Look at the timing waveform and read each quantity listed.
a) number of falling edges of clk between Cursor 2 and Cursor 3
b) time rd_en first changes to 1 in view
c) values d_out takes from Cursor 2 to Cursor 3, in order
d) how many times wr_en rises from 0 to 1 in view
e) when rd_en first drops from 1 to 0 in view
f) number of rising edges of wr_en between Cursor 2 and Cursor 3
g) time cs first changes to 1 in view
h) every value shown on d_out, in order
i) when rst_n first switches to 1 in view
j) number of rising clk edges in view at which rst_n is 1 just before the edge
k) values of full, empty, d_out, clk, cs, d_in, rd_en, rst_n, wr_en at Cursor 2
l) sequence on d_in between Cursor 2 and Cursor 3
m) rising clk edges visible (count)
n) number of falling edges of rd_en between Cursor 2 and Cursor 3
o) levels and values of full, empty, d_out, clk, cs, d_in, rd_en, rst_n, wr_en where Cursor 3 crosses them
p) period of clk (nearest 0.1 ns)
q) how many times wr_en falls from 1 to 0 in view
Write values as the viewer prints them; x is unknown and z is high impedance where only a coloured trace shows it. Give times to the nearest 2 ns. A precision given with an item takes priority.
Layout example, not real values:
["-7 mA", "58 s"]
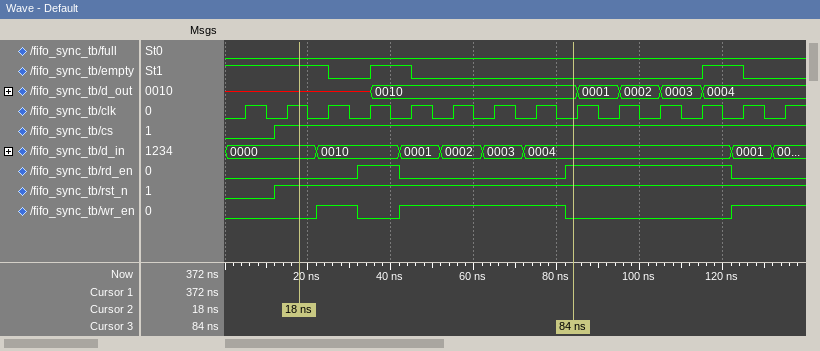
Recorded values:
["7", "32 ns", "x, 0010", "3", "42 ns", "2", "12 ns", "x, 0010, 0001, 0002, 0003, 0004", "12 ns", "13", "full=0, empty=1, d_out=x, clk=1, cs=1, d_in=0000, rd_en=0, rst_n=1, wr_en=0", "0000, 0010, 0001, 0002, 0003, 0004", "14", "1", "full=0, empty=0, d_out=0010, clk=0, cs=1, d_in=0004, rd_en=1, rst_n=1, wr_en=0", "10 ns", "2"]
